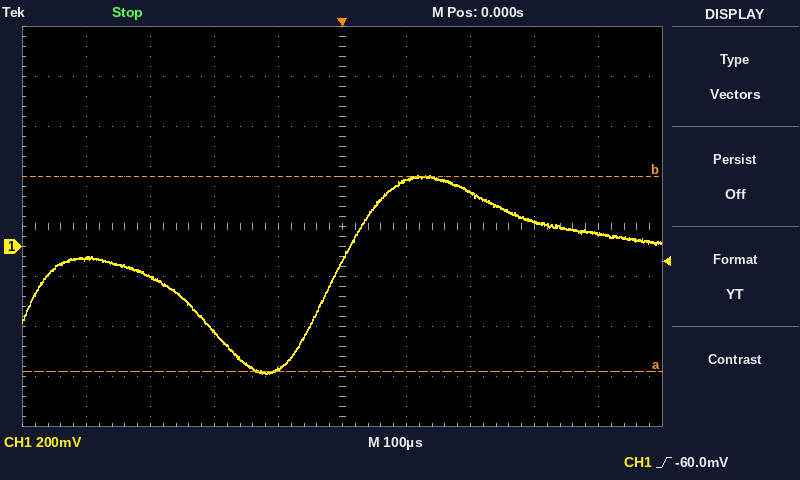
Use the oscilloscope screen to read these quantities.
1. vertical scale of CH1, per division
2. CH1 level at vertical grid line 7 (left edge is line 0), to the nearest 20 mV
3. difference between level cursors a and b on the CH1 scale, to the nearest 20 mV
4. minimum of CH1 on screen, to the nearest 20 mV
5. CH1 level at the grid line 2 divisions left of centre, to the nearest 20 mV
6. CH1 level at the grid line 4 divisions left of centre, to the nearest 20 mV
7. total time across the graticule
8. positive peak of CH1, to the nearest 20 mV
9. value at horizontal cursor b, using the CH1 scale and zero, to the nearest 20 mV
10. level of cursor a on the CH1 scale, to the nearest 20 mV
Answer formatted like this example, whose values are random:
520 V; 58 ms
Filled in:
200 mV; 220 mV; 780 mV; -500 mV; -340 mV; -40 mV; 1 ms; 280 mV; 280 mV; -500 mV
